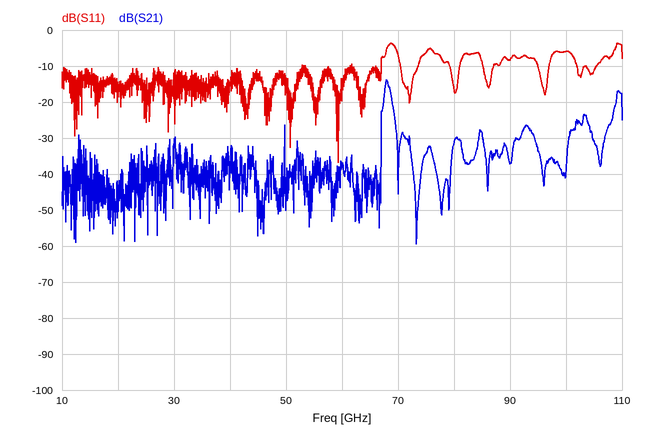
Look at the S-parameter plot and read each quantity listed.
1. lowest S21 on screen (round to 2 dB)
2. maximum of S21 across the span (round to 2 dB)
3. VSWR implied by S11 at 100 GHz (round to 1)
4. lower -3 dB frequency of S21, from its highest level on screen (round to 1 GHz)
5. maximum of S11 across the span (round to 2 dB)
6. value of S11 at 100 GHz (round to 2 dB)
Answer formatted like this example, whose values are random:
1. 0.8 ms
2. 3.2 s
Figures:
1. -60 dB
2. -14 dB
3. 3
4. 68 GHz
5. -4 dB
6. -6 dB
